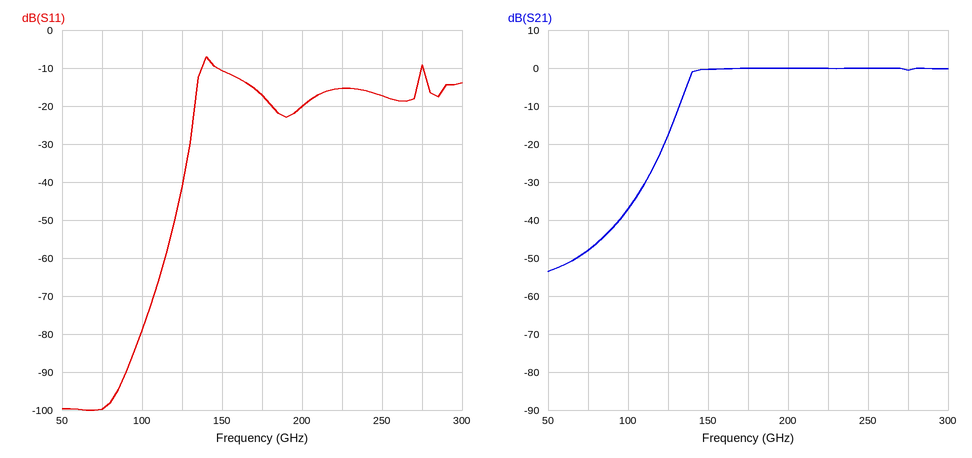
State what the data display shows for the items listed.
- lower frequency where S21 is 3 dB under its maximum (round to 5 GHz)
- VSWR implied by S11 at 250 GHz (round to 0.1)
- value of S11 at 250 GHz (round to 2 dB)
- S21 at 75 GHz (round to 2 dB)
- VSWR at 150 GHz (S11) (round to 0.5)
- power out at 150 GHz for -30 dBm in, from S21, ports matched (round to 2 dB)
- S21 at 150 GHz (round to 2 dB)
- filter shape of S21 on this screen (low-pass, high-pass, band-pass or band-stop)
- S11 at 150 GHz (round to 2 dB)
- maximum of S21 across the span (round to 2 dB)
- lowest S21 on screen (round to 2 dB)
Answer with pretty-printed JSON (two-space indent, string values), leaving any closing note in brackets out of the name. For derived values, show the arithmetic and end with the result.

{
  "lower frequency where S21 is 3 dB under its maximum": "140 GHz",
  "VSWR implied by S11 at 250 GHz": "|Γ| = 10^(-18/20) = 0.1259; VSWR = (1 + 0.1259)/(1 − 0.1259) ≈ 1.3",
  "value of S11 at 250 GHz": "-18 dB",
  "S21 at 75 GHz": "-48 dB",
  "VSWR at 150 GHz (S11)": "|Γ| = 10^(-10/20) = 0.3162; VSWR = (1 + 0.3162)/(1 − 0.3162) ≈ 1.92, so 2.0 to the nearest 0.5",
  "power out at 150 GHz for -30 dBm in, from S21, ports matched": "-30 dBm + (0 dB) = -30 dBm",
  "S21 at 150 GHz": "0 dB",
  "filter shape of S21 on this screen": "high-pass",
  "S11 at 150 GHz": "-10 dB",
  "maximum of S21 across the span": "0 dB",
  "lowest S21 on screen": "-54 dB"
}
